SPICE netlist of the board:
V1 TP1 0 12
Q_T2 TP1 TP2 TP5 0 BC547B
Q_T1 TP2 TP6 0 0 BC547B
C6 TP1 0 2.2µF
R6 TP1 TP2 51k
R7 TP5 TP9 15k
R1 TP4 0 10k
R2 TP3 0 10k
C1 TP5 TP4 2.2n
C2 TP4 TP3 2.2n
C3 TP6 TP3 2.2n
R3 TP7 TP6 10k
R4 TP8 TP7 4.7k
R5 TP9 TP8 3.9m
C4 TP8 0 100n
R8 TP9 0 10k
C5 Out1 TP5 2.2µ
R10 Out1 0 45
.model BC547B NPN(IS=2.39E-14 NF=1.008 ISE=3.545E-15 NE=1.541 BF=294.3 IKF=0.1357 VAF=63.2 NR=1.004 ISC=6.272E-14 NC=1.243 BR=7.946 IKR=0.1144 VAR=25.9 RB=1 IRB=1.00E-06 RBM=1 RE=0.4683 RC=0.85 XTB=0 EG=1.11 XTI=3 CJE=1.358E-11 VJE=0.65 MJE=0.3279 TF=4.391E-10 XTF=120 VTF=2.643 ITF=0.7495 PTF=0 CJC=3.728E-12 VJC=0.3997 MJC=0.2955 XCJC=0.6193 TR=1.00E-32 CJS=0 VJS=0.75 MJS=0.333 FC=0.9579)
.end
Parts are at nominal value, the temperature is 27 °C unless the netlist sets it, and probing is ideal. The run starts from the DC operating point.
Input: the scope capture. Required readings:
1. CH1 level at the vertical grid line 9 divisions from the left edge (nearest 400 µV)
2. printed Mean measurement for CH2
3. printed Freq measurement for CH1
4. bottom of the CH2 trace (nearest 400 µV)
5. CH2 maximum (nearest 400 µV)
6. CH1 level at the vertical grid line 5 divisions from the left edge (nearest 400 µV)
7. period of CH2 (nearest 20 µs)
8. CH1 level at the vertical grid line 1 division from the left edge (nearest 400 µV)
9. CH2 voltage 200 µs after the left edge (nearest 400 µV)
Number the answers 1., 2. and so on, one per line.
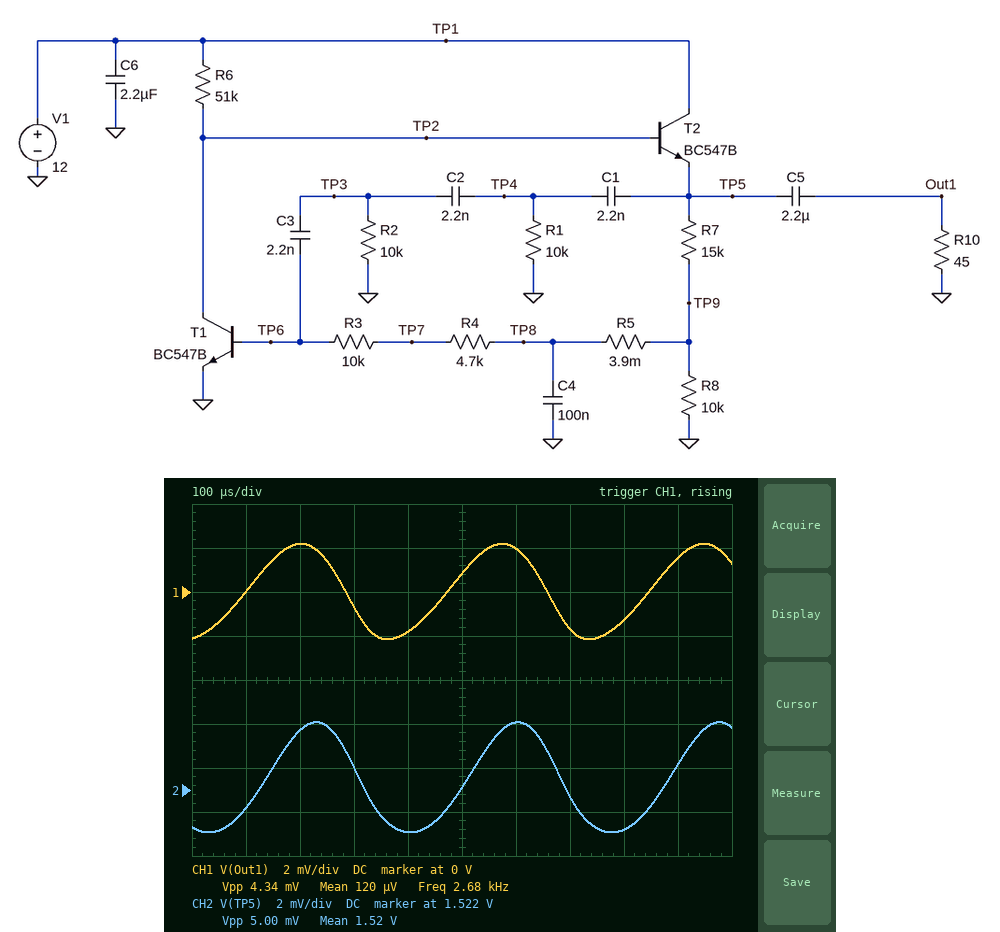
1. 1.6 mV
2. 1.52 V
3. 2.68 kHz
4. 1.5200 V
5. 1.5252 V
6. 800 µV
7. 380 µs
8. 0 V
9. 1.5248 V
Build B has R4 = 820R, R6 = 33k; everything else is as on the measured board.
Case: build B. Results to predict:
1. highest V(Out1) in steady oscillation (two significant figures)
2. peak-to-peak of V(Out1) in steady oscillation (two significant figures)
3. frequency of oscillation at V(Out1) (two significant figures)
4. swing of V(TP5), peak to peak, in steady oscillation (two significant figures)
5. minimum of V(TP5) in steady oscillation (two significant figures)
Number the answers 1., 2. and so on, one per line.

1. 2.0 mV
2. 4.0 mV
3. 3.1 kHz
4. 4.4 mV
5. 1.6 V
